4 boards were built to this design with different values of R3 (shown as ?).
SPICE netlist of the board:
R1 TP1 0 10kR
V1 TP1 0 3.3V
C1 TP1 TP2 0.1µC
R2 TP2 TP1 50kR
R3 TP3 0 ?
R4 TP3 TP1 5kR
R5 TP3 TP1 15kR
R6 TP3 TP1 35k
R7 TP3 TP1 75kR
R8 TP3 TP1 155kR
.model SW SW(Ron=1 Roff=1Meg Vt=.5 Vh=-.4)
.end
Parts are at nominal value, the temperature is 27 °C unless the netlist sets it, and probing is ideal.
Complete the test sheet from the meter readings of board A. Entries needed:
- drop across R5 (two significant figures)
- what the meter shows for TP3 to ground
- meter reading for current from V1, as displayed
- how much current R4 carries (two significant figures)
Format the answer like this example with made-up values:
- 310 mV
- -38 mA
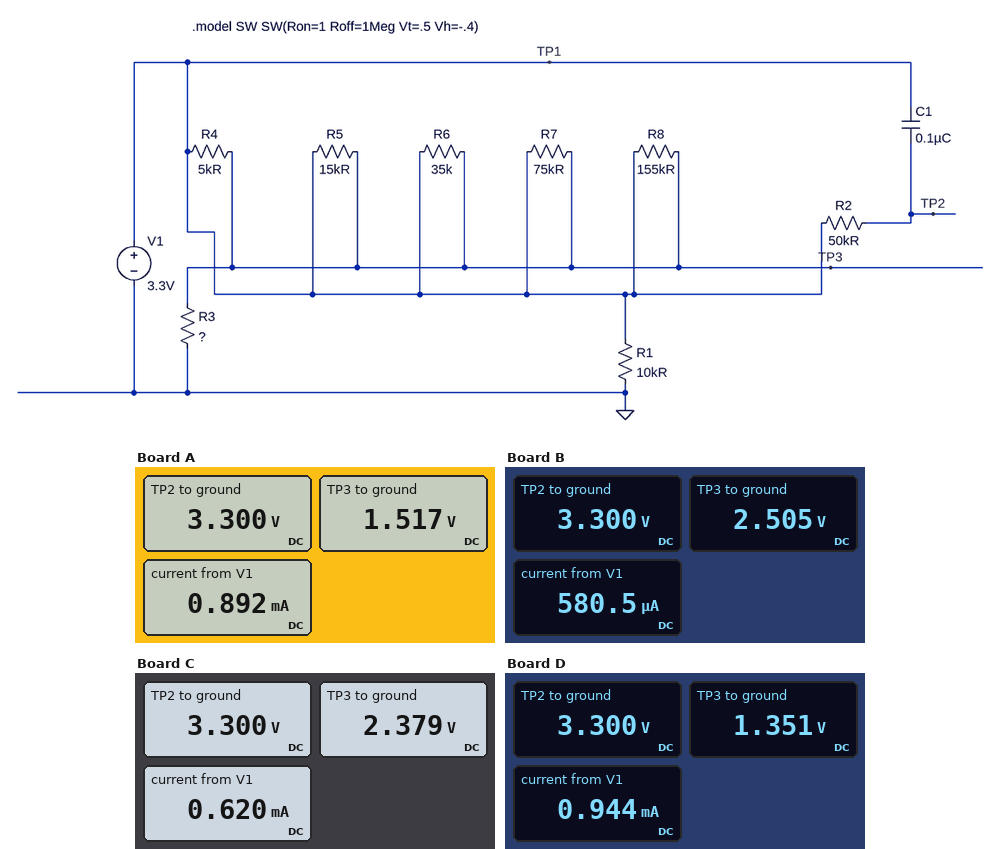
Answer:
- 1.8 V
- 1.517 V
- 0.892 mA
- 360 µA
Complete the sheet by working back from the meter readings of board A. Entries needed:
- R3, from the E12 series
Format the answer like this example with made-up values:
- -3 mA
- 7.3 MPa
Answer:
- 2.7 kΩ
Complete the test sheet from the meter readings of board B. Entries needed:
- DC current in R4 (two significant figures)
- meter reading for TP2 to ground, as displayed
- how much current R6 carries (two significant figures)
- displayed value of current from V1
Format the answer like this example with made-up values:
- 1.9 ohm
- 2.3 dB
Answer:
- 160 µA
- 3.300 V
- 23 µA
- 580.5 µA
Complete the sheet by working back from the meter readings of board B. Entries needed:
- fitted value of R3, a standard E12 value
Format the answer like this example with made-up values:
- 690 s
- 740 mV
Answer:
- 10 kΩ
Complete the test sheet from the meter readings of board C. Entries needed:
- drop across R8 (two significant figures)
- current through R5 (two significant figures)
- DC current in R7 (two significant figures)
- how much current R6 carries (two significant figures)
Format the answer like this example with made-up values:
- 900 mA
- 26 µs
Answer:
- 920 mV
- 61 µA
- 12 µA
- 26 µA
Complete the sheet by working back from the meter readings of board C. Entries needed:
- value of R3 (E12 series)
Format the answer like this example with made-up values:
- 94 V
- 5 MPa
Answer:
- 8.2 kΩ
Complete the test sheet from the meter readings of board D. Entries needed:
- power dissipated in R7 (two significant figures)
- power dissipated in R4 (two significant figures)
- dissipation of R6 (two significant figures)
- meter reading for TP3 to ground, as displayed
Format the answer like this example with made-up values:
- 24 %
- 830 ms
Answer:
- 51 µW
- 760 µW
- 110 µW
- 1.351 V
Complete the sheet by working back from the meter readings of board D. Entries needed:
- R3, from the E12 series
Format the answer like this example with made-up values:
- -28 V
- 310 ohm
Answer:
- 2.2 kΩ
